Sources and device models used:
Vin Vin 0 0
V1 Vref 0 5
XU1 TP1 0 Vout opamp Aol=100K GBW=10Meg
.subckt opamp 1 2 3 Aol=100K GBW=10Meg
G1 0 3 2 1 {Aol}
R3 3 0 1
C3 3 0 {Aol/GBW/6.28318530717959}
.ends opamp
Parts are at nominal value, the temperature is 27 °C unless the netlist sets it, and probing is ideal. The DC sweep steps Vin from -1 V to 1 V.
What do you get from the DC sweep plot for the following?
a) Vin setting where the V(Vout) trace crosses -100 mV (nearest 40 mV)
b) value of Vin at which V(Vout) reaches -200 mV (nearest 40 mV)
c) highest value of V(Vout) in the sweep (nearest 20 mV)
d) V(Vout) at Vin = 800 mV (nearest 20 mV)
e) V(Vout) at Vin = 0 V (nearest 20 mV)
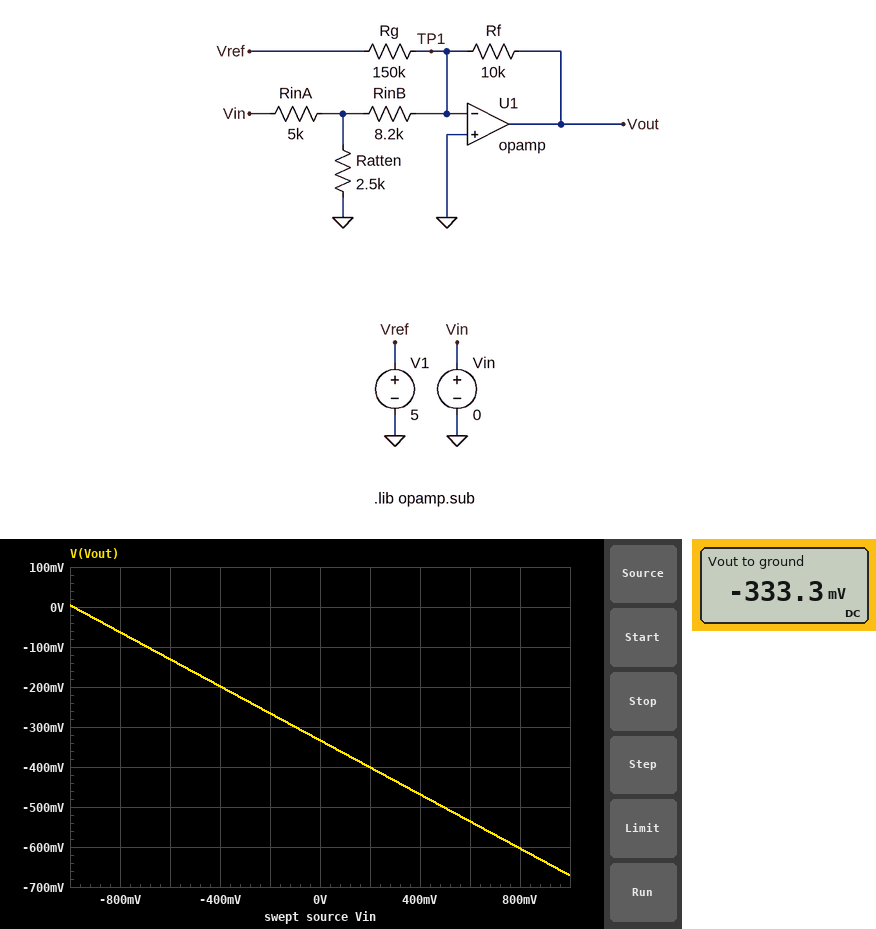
-680 mV
-400 mV
0 V
-600 mV
-340 mV
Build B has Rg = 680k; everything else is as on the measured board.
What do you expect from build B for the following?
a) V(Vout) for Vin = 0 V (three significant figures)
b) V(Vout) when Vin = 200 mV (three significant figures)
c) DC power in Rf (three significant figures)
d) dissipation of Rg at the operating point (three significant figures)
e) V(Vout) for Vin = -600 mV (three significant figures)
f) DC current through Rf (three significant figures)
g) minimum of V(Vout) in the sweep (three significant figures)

-73.5 mV
-141 mV
541 nW
36.8 µW
129 mV
7.35 µA
-411 mV
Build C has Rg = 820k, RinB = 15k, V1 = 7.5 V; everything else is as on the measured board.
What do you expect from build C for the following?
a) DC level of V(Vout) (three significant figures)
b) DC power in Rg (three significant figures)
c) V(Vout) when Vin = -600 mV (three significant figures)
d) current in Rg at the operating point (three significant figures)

-91.5 mV
68.6 µW
28.5 mV
9.15 µA
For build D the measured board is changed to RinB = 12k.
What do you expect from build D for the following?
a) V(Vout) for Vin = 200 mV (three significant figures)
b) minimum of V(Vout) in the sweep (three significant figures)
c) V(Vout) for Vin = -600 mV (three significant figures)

-382 mV
-577 mV
-187 mV
